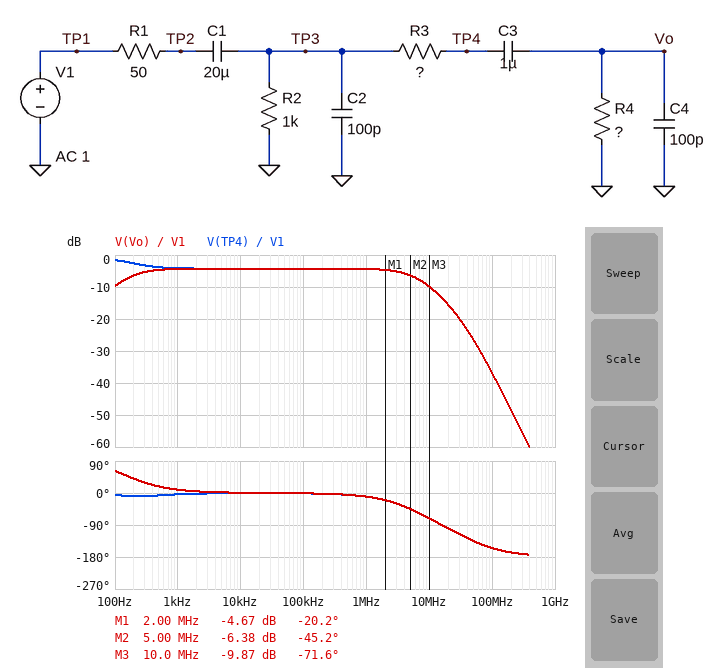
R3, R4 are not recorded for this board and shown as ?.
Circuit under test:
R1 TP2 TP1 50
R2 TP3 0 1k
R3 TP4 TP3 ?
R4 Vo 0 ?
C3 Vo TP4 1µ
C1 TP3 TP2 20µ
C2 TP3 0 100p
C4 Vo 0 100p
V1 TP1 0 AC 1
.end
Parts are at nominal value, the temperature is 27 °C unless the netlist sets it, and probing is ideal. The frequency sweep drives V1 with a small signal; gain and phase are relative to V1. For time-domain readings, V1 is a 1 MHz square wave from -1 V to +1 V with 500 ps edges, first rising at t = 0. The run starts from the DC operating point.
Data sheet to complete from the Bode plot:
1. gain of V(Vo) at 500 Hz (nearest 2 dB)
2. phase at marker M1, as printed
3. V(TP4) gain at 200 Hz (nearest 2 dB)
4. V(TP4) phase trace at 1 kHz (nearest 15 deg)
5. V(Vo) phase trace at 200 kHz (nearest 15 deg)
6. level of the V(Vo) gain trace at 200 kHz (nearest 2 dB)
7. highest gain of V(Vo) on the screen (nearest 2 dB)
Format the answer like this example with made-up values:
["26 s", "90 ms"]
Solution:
["-4 dB", "-20.2 deg", "-2 dB", "0 deg", "0 deg", "-4 dB", "-4 dB"]
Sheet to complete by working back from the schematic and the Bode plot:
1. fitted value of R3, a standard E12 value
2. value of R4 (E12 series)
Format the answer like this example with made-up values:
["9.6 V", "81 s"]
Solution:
["330 Ω", "680 Ω"]
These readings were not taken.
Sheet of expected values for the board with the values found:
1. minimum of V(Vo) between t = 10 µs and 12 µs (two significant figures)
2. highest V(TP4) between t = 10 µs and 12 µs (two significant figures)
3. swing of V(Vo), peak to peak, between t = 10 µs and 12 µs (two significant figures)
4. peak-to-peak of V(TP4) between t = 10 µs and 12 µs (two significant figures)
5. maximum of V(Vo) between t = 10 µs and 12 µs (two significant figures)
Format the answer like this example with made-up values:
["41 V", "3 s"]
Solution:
["-7.6 mV", "1.2 V", "1.2 V", "1.2 V", "1.2 V"]
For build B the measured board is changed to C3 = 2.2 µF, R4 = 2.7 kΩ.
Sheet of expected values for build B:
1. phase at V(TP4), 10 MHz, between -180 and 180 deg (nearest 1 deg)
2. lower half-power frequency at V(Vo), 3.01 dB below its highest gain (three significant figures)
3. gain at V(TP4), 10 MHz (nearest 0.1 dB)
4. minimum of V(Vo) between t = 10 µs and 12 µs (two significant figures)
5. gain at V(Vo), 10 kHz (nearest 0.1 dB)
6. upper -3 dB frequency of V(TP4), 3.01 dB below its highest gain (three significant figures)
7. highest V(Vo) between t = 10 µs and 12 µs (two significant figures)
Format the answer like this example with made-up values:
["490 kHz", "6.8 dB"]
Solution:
["-79 deg", "28.3 Hz", "-9.2 dB", "-2.1 mV", "-1.6 dB", "4.65 MHz", "1.7 V"]
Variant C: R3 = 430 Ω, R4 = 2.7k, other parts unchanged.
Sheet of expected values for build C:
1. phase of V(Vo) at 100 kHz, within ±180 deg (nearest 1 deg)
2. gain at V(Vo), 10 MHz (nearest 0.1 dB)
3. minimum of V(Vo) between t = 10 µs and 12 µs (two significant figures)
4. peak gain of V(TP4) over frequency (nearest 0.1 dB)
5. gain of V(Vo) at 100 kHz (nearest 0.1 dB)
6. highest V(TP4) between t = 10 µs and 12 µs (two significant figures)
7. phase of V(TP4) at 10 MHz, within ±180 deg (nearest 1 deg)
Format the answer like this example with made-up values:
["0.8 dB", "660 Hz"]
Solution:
["-2 deg", "-11.0 dB", "-3.6 mV", "-1.3 dB", "-1.8 dB", "1.6 V", "-84 deg"]
